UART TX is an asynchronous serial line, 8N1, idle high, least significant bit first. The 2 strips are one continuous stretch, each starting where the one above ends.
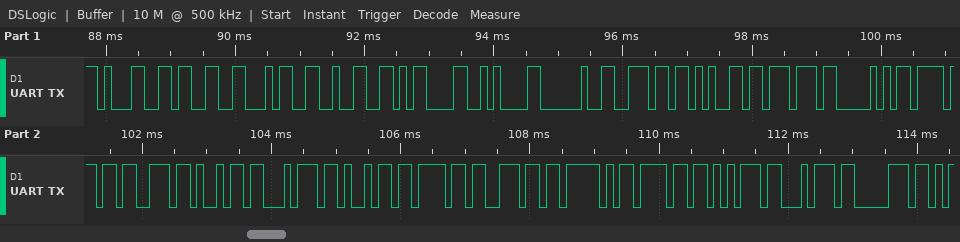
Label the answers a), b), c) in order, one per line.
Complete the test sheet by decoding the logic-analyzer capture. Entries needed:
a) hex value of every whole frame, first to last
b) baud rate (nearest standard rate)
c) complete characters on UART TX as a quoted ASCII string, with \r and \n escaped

a) 31 33 34 32 0D 0A 20 6E 65 77 50 6F 73 69 74 69 6F 6E 5F 6F 75 74 70
b) 9600 baud
c) "1342\r\n newPosition_outp"
